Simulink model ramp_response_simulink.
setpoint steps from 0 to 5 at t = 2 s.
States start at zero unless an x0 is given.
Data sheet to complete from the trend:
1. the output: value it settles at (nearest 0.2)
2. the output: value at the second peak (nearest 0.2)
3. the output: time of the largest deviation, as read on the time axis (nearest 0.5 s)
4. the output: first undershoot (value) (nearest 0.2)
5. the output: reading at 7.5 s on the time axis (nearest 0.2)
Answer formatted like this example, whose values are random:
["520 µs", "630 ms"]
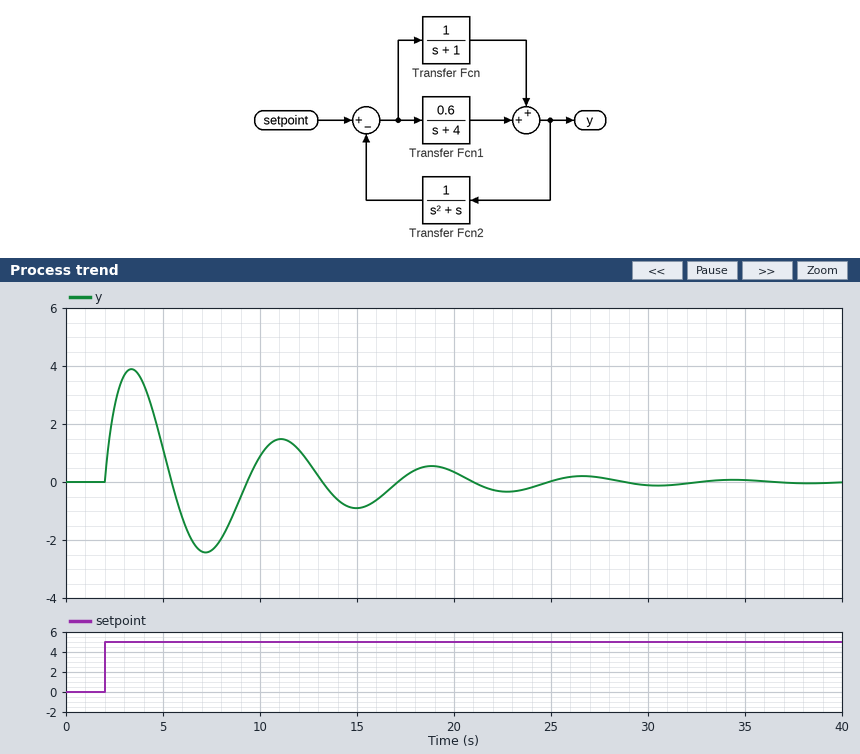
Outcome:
["0.0", "1.4", "3.5 s", "-2.4", "-2.4"]
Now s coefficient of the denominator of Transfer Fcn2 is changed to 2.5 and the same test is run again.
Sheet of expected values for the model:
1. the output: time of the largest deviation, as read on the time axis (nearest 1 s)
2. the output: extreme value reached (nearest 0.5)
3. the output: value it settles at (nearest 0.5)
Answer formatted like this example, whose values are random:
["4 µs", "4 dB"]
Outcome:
["4 s", "4.0", "0.0"]
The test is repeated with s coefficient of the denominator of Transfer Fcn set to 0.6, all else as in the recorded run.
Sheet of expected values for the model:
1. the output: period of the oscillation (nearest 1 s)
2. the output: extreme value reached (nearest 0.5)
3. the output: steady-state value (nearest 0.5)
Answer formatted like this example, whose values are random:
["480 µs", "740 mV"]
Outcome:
["7 s", "4.5", "0.0"]
